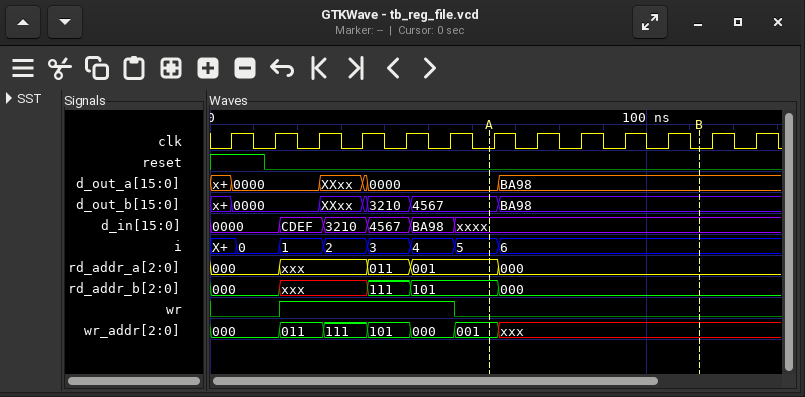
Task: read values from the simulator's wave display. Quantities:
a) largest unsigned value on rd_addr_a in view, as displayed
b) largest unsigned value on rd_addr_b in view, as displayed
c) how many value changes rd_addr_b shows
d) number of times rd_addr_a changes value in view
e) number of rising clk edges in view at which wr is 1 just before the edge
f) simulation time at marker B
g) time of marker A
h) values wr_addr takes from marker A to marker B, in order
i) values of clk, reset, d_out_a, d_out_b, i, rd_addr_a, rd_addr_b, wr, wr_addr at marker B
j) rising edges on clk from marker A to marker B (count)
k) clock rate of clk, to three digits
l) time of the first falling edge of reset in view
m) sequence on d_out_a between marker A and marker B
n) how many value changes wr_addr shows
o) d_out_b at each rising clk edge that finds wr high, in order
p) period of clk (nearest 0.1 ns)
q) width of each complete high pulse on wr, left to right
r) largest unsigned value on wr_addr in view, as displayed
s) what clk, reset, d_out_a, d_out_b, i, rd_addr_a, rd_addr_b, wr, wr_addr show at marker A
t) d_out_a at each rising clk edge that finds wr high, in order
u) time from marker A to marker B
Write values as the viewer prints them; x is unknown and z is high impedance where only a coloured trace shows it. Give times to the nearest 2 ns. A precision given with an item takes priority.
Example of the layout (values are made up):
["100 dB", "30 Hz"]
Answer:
["011", "111", "4", "4", "4", "112 ns", "64 ns", "001, xxx", "clk=0, reset=0, d_out_a=BA98, d_out_b=BA98, i=6, rd_addr_a=000, rd_addr_b=000, wr=0, wr_addr=xxx", "5", "100 MHz", "12 ns", "0000, BA98", "6", "0000, XXxx, 3210, 4567", "10 ns", "40 ns", "111", "clk=0, reset=0, d_out_a=0000, d_out_b=4567, i=5, rd_addr_a=001, rd_addr_b=101, wr=0, wr_addr=001", "0000, XXxx, 0000, 0000", "48 ns"]
